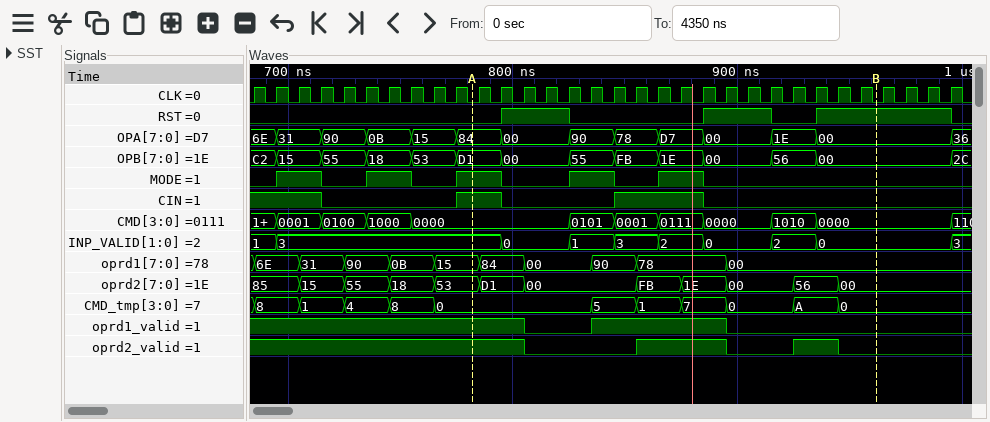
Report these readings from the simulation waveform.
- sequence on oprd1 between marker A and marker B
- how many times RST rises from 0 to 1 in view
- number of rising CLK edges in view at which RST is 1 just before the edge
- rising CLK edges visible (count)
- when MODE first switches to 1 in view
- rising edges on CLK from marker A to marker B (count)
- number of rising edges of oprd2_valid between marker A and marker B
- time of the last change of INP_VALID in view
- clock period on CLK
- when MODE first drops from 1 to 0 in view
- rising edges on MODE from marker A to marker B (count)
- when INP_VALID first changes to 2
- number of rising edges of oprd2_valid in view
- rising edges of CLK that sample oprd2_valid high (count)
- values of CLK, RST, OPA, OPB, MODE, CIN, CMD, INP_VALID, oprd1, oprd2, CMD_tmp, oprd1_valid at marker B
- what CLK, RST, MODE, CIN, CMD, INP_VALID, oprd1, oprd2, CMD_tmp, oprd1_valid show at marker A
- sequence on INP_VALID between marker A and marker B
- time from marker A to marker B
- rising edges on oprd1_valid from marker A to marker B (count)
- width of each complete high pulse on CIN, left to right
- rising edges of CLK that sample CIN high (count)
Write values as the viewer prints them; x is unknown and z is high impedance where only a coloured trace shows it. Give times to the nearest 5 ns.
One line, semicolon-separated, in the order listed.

15, 84, 00, 90, 78, 00; 3; 12; 32; 695 ns; 18; 2; 995 ns; 10 ns; 715 ns; 2; 865 ns; 2; 19; CLK=0, RST=1, OPA=00, OPB=00, MODE=0, CIN=0, CMD=0000, INP_VALID=0, oprd1=00, oprd2=00, CMD_tmp=0, oprd1_valid=0; CLK=0, RST=0, MODE=1, CIN=1, CMD=0000, INP_VALID=3, oprd1=15, oprd2=53, CMD_tmp=0, oprd1_valid=1; 3, 0, 1, 3, 2, 0, 2, 0; 180 ns; 1; 20 ns, 40 ns; 10
